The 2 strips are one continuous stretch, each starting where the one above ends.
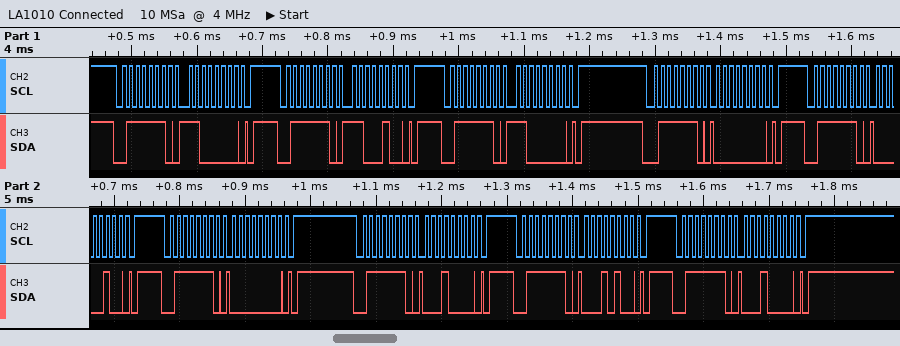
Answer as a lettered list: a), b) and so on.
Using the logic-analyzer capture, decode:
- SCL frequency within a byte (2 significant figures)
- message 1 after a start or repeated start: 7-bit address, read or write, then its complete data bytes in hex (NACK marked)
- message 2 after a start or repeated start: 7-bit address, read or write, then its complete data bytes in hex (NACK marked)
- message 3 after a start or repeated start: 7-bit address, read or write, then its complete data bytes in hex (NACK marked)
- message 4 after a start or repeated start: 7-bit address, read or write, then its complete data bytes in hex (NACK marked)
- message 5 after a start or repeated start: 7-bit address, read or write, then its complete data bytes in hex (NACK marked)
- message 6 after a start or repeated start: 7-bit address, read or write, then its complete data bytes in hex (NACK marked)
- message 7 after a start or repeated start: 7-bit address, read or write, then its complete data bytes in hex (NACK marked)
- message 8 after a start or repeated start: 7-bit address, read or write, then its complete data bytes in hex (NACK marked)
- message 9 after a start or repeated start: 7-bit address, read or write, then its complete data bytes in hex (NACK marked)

a) 100 kHz
b) 0x3F write: C0
c) 0x3F write: C4
d) 0x3F write: C0
e) 0x3F write: 00
f) 0x3F write: 04
g) 0x3F write: 00
h) 0x3F write: 10
i) 0x3F write: 14
j) 0x3F write: 10
